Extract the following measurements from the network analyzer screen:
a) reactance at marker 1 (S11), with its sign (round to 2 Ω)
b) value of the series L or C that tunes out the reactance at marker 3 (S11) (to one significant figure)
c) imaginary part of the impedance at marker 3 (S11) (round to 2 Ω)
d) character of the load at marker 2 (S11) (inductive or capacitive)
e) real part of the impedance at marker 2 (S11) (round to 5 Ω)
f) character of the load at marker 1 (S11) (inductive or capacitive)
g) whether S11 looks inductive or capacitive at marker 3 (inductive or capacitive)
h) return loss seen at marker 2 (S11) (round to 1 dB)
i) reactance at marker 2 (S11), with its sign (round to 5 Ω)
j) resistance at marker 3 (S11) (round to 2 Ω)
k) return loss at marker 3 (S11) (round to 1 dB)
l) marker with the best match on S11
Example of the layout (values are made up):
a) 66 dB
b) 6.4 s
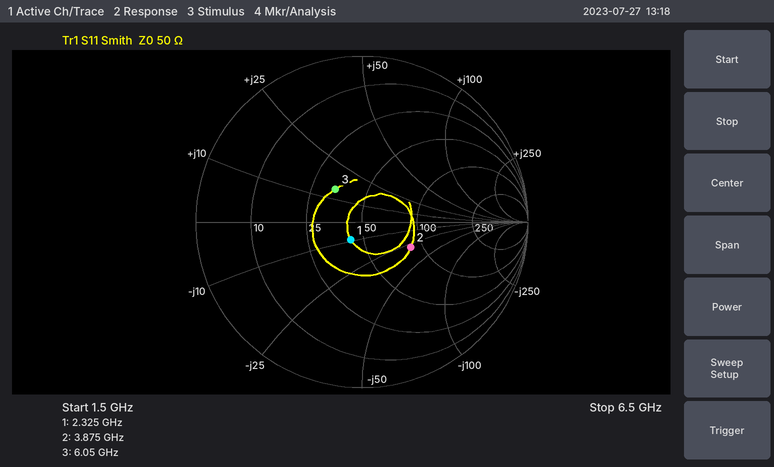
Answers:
a) -10 Ω
b) 2 pF
c) +14 Ω
d) capacitive
e) 85 Ω
f) capacitive
g) inductive
h) 10 dB
i) -30 Ω
j) 34 Ω
k) 12 dB
l) marker 1
